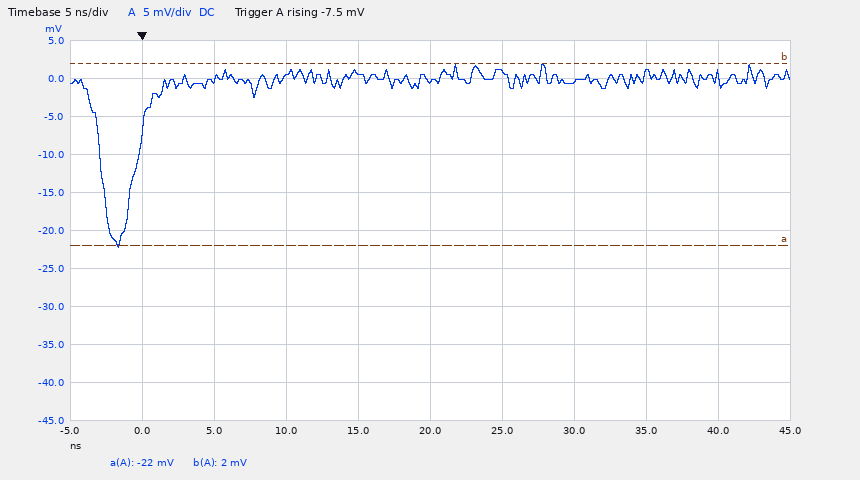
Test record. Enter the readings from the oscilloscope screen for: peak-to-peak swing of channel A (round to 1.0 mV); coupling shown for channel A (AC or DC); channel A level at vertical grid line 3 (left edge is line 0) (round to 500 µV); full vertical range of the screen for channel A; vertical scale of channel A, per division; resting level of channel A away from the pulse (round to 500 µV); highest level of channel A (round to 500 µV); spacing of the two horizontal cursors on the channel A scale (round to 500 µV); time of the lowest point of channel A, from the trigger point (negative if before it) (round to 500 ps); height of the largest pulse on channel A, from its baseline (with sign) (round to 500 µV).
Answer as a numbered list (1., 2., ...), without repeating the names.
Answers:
1. 24.0 mV
2. DC
3. 500 µV
4. 50 mV
5. 5 mV
6. 0.0 mV
7. 2.0 mV
8. 24.0 mV
9. -1.5 ns
10. -22.0 mV
